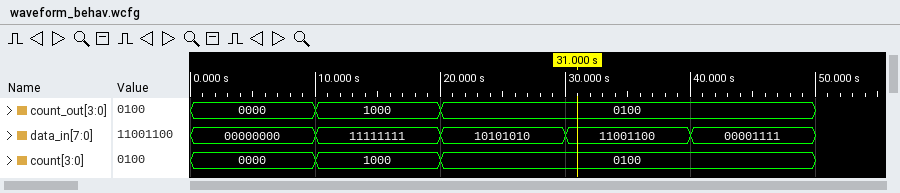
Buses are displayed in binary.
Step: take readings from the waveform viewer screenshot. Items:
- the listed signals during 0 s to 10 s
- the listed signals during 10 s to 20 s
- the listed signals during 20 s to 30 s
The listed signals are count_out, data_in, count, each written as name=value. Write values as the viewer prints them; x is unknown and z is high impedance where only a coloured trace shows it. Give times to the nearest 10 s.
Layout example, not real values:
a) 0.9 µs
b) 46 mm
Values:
a) count_out=0000, data_in=00000000, count=0000
b) count_out=1000, data_in=11111111, count=1000
c) count_out=0100, data_in=10101010, count=0100
